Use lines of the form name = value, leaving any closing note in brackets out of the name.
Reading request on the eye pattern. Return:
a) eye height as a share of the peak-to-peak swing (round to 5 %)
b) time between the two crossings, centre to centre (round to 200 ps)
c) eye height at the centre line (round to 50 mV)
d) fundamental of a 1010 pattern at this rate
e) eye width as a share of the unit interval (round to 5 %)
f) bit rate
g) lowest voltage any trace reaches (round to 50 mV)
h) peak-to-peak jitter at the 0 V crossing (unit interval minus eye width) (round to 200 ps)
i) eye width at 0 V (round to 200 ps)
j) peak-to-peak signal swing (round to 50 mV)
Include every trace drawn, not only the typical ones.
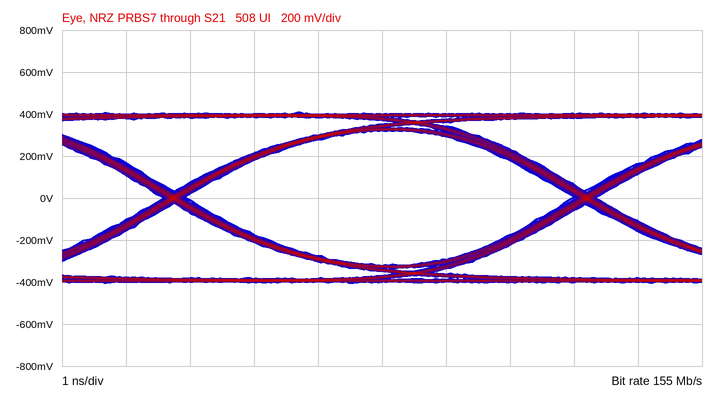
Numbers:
eye height as a share of the peak-to-peak swing = 80 %
time between the two crossings, centre to centre = 6.4 ns
eye height at the centre line = 650 mV
fundamental of a 1010 pattern at this rate = 77.5 MHz
eye width as a share of the unit interval = 95 %
bit rate = 155 Mb/s
lowest voltage any trace reaches = -400 mV
peak-to-peak jitter at the 0 V crossing (unit interval minus eye width) = 400 ps
eye width at 0 V = 6.0 ns
peak-to-peak signal swing = 800 mV
